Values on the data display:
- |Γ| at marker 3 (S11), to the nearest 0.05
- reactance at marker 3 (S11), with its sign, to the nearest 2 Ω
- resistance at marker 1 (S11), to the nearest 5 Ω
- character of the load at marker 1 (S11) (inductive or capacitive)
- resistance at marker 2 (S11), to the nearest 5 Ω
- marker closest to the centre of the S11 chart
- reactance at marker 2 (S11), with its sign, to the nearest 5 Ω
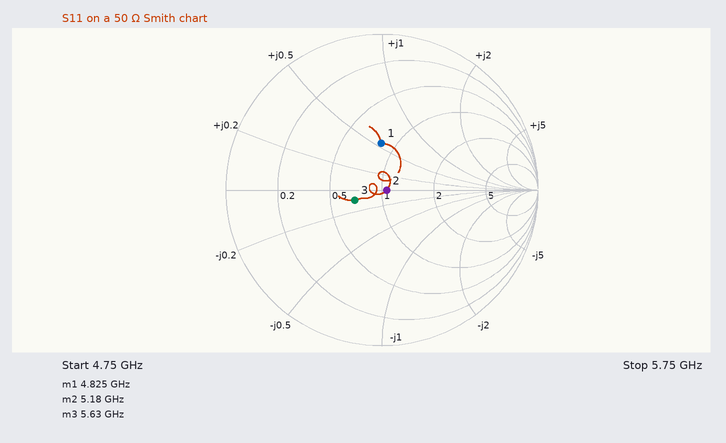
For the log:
0.20
-4 Ω
40 Ω
inductive
55 Ω
marker 2
0 Ω
